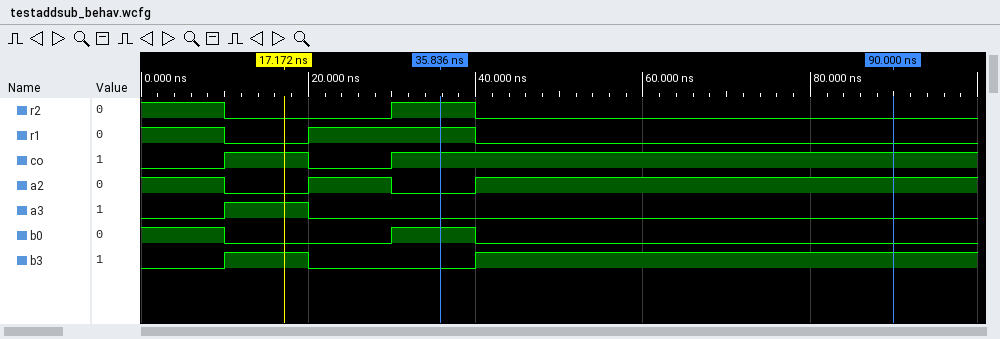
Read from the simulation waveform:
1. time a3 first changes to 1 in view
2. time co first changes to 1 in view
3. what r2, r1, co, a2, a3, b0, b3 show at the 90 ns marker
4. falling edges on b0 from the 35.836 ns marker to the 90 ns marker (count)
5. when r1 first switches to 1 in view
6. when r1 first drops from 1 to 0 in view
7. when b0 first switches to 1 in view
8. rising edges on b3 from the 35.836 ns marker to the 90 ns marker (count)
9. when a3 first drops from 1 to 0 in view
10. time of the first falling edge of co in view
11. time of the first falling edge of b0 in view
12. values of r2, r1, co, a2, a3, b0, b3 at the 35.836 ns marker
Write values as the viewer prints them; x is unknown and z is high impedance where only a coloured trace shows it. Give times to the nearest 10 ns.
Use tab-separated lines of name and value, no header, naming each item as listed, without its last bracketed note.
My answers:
time a3 first changes to 1 in view	10 ns
time co first changes to 1 in view	10 ns
what r2, r1, co, a2, a3, b0, b3 show at the 90 ns marker	r2=0, r1=0, co=1, a2=1, a3=0, b0=0, b3=1
falling edges on b0 from the 35.836 ns marker to the 90 ns marker	1
when r1 first switches to 1 in view	20 ns
when r1 first drops from 1 to 0 in view	10 ns
when b0 first switches to 1 in view	30 ns
rising edges on b3 from the 35.836 ns marker to the 90 ns marker	1
when a3 first drops from 1 to 0 in view	20 ns
time of the first falling edge of co in view	20 ns
time of the first falling edge of b0 in view	10 ns
values of r2, r1, co, a2, a3, b0, b3 at the 35.836 ns marker	r2=1, r1=1, co=1, a2=0, a3=0, b0=1, b3=0
